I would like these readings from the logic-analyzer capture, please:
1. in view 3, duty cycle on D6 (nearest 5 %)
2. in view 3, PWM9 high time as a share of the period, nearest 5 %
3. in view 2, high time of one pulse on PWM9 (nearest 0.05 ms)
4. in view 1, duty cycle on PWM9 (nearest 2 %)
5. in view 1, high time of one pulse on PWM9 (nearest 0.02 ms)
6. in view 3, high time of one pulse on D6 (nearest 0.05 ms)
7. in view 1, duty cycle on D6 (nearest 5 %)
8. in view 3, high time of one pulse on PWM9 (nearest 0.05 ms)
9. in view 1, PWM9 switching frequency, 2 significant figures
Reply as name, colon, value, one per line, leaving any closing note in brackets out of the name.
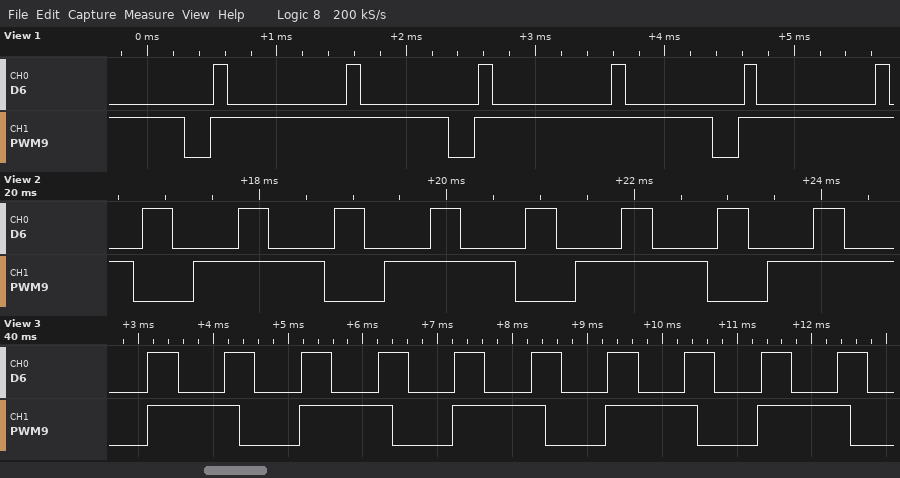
in view 3, duty cycle on D6: 40 %
in view 3, PWM9 high time as a share of the period, nearest 5 %: 60 %
in view 2, high time of one pulse on PWM9: 1.40 ms
in view 1, duty cycle on PWM9: 90 %
in view 1, high time of one pulse on PWM9: 1.84 ms
in view 3, high time of one pulse on D6: 0.40 ms
in view 1, duty cycle on D6: 10 %
in view 3, high time of one pulse on PWM9: 1.25 ms
in view 1, PWM9 switching frequency, 2 significant figures: 490 Hz
